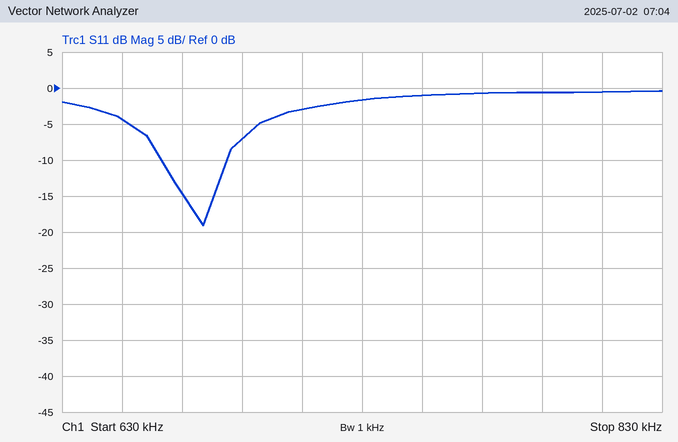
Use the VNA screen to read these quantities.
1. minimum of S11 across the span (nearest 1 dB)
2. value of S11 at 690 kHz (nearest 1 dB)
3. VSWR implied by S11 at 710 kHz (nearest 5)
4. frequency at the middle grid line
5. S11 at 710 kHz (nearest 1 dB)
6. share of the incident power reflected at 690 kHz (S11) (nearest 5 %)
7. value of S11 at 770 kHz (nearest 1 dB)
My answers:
-19 dB
-7 dB
5
730 kHz
-3 dB
20 %
-1 dB
